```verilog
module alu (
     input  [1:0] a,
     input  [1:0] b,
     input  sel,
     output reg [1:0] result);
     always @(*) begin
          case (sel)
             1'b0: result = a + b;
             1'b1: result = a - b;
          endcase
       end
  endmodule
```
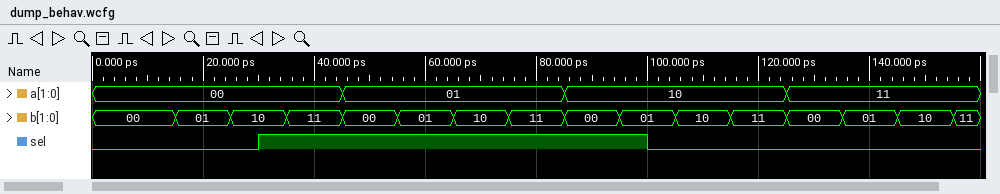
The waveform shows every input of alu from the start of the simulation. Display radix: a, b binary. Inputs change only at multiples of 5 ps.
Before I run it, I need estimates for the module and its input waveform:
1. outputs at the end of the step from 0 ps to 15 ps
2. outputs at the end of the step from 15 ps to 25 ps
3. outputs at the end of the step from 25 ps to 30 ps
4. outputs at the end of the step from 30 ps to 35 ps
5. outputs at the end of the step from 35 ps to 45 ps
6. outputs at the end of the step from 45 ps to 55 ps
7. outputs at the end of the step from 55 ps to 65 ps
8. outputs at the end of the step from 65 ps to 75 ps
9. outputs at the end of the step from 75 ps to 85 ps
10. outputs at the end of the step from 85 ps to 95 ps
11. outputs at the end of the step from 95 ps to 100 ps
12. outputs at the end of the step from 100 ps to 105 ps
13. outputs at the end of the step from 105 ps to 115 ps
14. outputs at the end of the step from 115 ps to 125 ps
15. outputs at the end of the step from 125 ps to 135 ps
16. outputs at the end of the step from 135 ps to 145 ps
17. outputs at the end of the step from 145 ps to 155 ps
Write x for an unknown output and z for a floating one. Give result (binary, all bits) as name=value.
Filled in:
result=00
result=01
result=10
result=10
result=01
result=01
result=00
result=11
result=10
result=10
result=01
result=11
result=00
result=01
result=11
result=00
result=01
